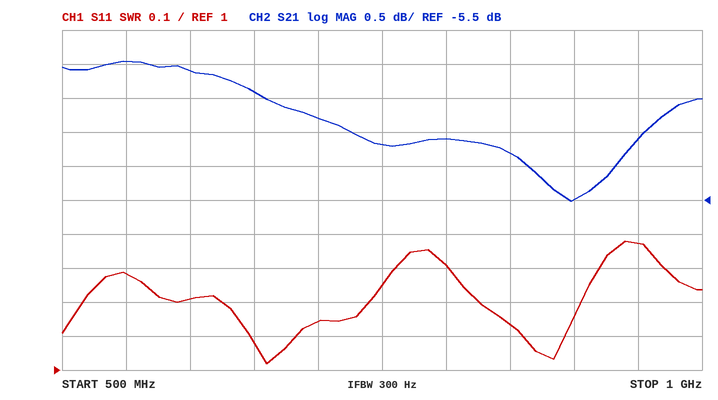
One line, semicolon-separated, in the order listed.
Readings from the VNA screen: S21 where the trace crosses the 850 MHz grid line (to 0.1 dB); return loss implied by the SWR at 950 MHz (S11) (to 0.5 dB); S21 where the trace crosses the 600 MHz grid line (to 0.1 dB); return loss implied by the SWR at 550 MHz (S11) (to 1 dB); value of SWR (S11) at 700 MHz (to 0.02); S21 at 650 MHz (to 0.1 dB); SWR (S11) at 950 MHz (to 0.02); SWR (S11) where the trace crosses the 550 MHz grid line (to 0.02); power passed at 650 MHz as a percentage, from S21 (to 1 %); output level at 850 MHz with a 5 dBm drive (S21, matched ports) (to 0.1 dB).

-4.8 dB; 16.0 dB; -3.6 dB; 18 dB; 1.14; -3.9 dB; 1.38; 1.28; 41 %; 0.2 dBm
